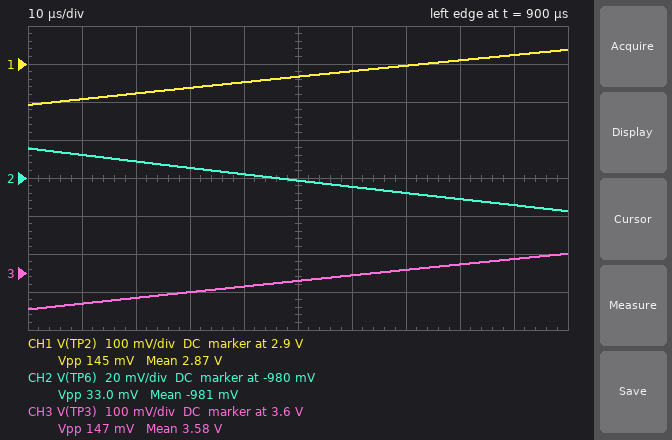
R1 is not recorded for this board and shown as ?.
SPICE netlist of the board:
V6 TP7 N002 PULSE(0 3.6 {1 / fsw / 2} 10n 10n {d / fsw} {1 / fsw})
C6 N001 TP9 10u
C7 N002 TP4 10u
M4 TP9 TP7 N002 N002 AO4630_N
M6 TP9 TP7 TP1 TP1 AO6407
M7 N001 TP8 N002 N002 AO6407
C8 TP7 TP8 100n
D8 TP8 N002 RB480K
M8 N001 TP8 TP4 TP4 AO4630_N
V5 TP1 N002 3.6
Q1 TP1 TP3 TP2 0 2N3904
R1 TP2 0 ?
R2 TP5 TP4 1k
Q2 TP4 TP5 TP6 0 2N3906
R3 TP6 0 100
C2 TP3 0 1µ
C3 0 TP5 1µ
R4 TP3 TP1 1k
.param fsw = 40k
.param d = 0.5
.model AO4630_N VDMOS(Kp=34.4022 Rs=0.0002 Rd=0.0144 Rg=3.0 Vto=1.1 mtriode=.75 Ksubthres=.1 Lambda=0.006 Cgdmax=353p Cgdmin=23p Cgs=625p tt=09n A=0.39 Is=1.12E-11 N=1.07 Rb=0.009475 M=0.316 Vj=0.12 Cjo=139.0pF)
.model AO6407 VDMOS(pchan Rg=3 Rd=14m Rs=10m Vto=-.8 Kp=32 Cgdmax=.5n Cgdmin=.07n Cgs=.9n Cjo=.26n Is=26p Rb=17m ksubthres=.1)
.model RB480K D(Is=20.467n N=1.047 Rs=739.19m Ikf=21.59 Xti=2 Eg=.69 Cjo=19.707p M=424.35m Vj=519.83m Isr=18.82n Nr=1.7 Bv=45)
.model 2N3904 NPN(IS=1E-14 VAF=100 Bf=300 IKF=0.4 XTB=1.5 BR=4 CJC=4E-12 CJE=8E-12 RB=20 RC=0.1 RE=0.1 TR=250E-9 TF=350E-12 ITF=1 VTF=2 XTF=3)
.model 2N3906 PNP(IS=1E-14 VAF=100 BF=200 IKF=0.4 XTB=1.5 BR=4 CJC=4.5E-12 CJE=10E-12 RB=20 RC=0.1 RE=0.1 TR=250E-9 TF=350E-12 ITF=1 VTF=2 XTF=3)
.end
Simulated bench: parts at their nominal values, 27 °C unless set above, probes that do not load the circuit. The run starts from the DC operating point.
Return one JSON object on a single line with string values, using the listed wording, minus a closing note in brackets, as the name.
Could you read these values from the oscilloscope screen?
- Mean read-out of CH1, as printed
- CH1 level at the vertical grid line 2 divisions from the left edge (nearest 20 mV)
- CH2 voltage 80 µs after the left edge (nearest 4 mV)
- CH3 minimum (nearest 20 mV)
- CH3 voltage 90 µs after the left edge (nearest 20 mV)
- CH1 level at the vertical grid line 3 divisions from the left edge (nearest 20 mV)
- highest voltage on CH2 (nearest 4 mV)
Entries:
{"Mean read-out of CH1, as printed": "2.87 V", "CH1 level at the vertical grid line 2 divisions from the left edge": "2.82 V", "CH2 voltage 80 µs after the left edge": "-992 mV", "CH3 minimum": "3.50 V", "CH3 voltage 90 µs after the left edge": "3.64 V", "CH1 level at the vertical grid line 3 divisions from the left edge": "2.84 V", "highest voltage on CH2": "-964 mV"}
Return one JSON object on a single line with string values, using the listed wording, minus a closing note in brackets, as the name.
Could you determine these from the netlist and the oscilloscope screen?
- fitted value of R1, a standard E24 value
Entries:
{"fitted value of R1, a standard E24 value": "330 Ω"}
